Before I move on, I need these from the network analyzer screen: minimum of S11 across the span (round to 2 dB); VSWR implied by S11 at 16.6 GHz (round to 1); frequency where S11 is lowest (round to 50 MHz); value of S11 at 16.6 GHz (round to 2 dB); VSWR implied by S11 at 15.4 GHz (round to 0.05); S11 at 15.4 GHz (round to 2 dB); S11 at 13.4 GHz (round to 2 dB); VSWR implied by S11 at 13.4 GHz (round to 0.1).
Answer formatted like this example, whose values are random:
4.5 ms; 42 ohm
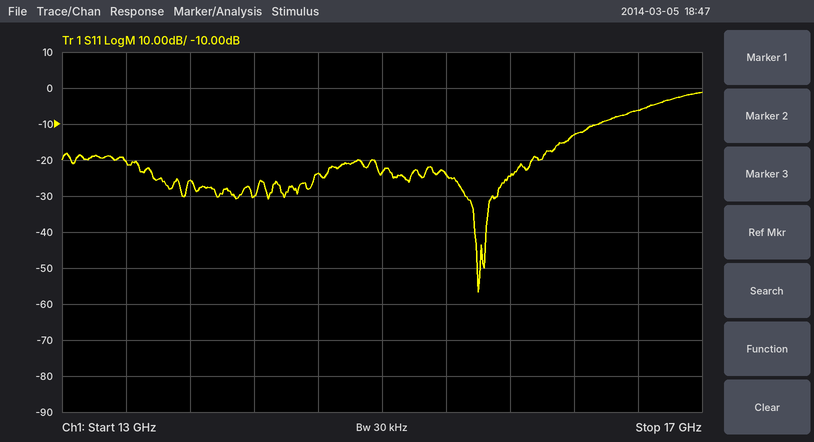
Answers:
-56 dB; 3; 15.60 GHz; -6 dB; 1.15; -24 dB; -20 dB; 1.2
